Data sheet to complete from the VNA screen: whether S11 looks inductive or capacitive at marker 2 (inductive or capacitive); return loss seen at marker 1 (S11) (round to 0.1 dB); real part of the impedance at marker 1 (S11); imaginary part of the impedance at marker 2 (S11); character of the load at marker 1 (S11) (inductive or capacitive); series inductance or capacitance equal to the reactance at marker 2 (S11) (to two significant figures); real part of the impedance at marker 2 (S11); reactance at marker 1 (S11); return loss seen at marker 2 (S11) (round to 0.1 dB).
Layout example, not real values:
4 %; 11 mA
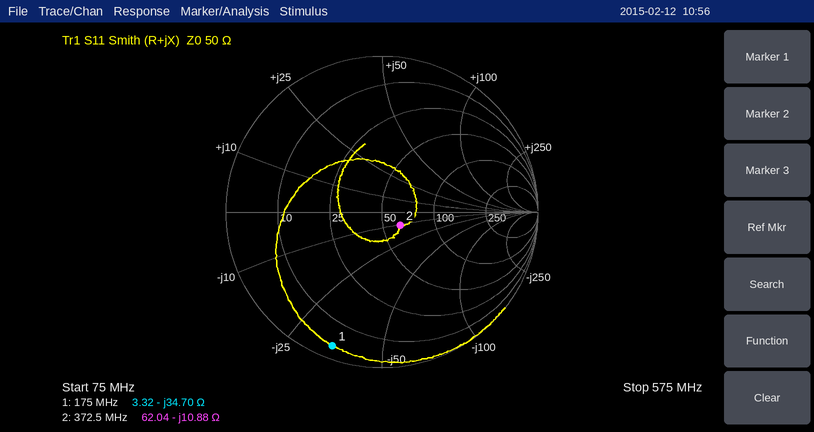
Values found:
capacitive; 0.8 dB; 3.32 Ω; -10.88 Ω; capacitive; 39 pF; 62.04 Ω; -34.70 Ω; 16.8 dB
